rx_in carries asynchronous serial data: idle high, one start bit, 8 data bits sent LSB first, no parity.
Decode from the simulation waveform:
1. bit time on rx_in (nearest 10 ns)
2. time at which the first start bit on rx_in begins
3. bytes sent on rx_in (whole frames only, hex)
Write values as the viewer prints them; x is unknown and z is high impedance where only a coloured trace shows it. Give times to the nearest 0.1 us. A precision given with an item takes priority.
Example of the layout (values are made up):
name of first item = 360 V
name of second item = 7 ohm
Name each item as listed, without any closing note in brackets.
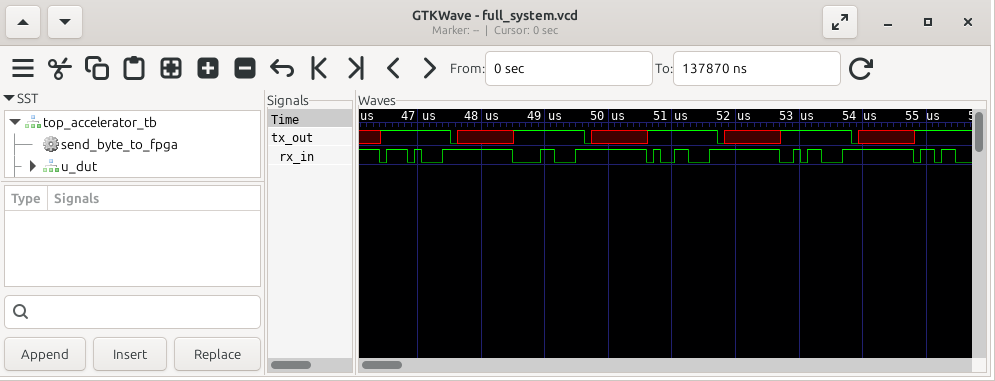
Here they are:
bit time on rx_in = 110 ns
time at which the first start bit on rx_in begins = 46.4 us
bytes sent on rx_in = 17, 18, 19, 1A
